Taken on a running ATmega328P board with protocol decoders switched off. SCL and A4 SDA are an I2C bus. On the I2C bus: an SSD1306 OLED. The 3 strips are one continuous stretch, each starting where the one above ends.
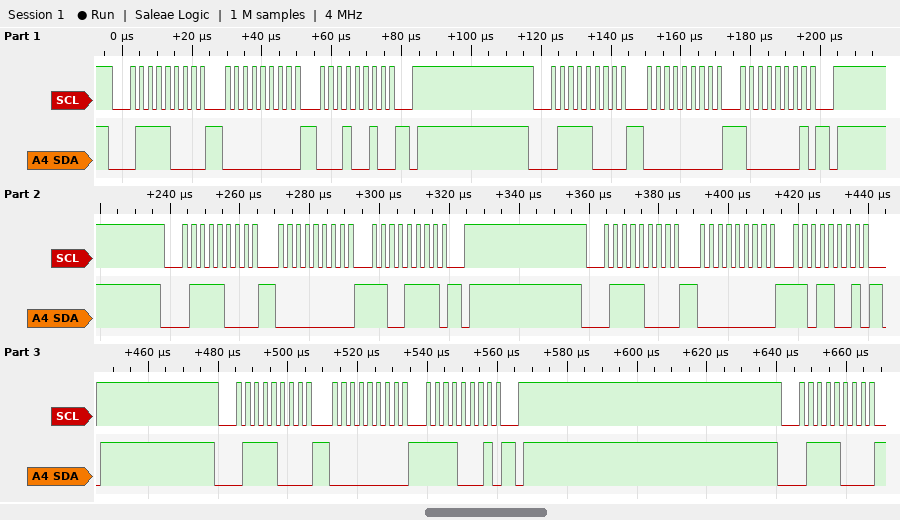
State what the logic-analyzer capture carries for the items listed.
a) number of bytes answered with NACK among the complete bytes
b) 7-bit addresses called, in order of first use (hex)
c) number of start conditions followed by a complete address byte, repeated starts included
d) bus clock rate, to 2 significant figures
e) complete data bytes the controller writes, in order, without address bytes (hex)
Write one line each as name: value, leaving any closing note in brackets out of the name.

number of bytes answered with NACK among the complete bytes: 0
7-bit addresses called, in order of first use: 0x3C
number of start conditions followed by a complete address byte, repeated starts included: 6
bus clock rate, to 2 significant figures: 400 kHz
complete data bytes the controller writes, in order, without address bytes: 00 12 00 81 00 CF 00 D9 00 F1
